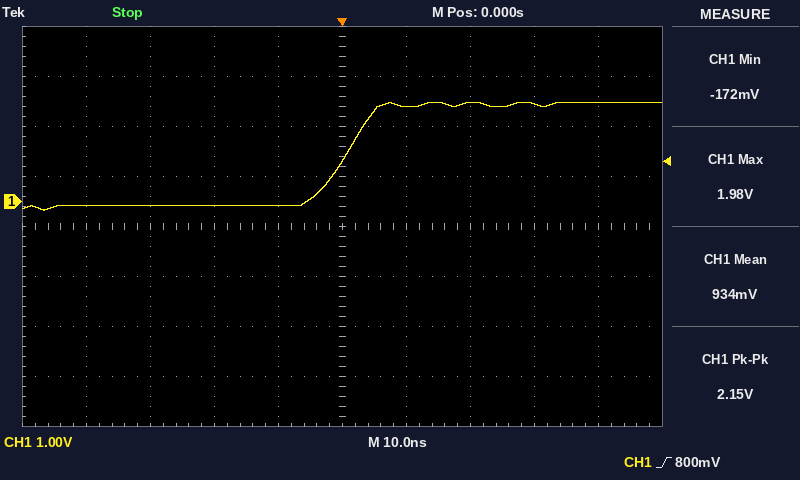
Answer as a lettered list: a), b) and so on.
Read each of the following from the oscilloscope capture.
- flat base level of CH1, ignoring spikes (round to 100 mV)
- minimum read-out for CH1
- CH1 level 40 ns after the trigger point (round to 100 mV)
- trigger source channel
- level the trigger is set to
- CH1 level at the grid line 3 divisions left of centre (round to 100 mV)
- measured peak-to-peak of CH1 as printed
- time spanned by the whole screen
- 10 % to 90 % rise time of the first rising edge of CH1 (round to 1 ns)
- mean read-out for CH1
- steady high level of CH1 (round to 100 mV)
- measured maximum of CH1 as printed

a) -100 mV
b) -172 mV
c) 2.0 V
d) CH1
e) 800 mV
f) -100 mV
g) 2.15 V
h) 100 ns
i) 9 ns
j) 934 mV
k) 2.0 V
l) 1.98 V
